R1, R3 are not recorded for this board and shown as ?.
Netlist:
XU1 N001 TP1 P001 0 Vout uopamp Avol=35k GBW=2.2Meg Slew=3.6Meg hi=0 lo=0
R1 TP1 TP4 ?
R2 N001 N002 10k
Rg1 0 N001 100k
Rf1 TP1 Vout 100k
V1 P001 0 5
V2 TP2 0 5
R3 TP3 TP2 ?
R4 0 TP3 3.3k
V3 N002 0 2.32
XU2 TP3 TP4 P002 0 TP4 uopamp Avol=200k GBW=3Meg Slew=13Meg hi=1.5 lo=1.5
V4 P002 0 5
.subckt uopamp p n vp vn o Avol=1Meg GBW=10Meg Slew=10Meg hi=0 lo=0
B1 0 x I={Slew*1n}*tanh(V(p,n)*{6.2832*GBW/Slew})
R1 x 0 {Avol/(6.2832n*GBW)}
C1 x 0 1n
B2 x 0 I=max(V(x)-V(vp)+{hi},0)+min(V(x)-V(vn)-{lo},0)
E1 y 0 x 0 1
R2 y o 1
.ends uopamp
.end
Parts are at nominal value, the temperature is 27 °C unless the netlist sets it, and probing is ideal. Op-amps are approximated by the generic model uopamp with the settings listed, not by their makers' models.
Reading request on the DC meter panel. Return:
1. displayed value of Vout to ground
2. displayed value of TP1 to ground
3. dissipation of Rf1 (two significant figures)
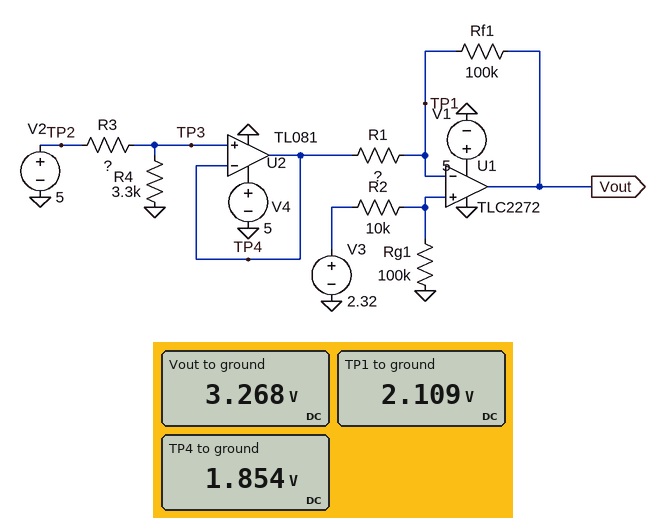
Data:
3.268 V
2.109 V
13 µW
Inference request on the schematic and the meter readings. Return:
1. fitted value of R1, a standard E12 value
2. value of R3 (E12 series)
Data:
22 kΩ
5.6 kΩ
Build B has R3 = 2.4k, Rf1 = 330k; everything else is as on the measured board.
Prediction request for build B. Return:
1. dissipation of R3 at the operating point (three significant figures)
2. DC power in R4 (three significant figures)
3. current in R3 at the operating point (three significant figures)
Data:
1.85 mW
2.54 mW
877 µA
